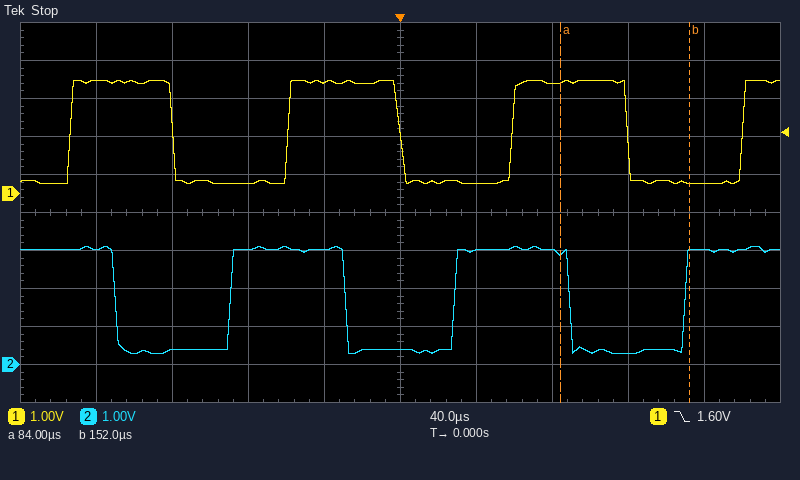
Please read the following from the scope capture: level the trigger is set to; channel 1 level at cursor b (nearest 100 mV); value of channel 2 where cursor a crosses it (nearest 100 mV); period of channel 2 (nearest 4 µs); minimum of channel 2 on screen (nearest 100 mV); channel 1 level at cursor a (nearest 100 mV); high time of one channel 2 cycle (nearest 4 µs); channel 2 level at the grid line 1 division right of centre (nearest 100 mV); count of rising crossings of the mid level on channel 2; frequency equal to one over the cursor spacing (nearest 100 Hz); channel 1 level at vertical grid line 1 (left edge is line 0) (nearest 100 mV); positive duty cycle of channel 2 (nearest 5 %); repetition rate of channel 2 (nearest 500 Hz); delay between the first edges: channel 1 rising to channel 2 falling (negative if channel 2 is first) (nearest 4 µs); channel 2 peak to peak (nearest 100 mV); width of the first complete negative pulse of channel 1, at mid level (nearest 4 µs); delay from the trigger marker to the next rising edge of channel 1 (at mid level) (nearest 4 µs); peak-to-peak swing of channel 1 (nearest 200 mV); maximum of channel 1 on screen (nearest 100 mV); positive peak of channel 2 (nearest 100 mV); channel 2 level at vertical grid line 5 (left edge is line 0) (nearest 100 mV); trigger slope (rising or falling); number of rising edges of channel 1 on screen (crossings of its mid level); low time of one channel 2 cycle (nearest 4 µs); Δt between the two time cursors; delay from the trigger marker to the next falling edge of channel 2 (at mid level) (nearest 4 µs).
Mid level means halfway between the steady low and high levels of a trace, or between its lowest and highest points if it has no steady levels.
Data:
1.60 V
300 mV
2.9 V
120 µs
300 mV
2.9 V
60 µs
3.0 V
3
14.7 kHz
3.0 V
50 %
8.5 kHz
+24 µs
2.8 V
60 µs
60 µs
2.8 V
3.0 V
3.1 V
400 mV
falling
4
60 µs
68 µs
88 µs
